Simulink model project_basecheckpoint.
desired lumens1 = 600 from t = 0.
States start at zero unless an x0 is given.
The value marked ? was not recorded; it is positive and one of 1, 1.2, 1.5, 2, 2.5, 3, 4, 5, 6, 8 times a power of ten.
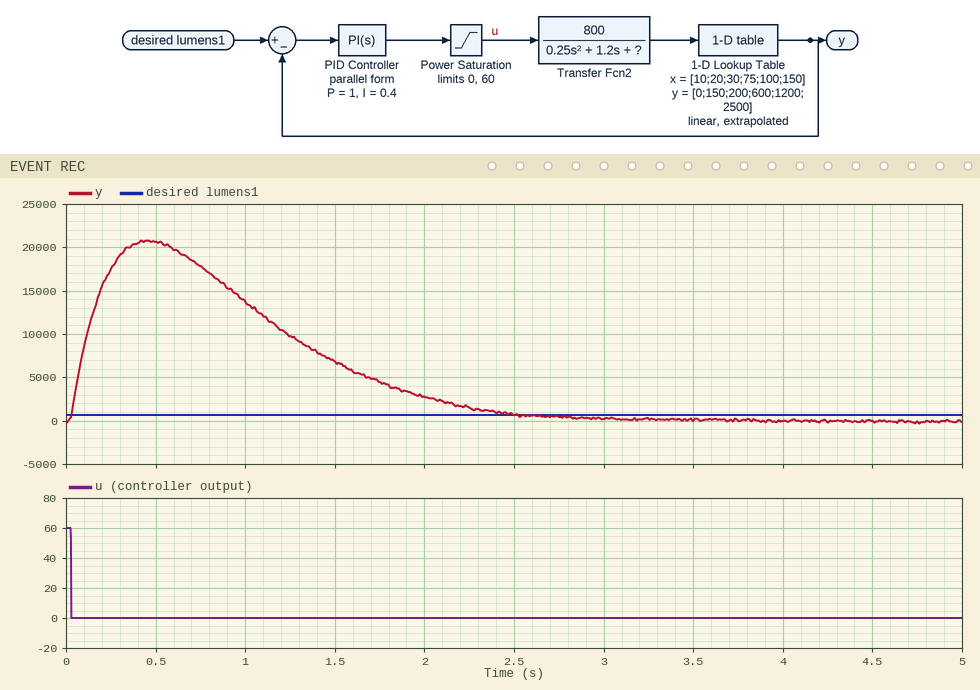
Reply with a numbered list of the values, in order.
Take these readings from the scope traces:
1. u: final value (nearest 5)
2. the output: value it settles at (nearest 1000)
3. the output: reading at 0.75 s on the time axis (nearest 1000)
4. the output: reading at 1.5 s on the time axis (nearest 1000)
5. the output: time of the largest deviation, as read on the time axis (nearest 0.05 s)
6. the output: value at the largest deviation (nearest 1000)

1. 0
2. 0
3. 18000
4. 7000
5. 0.45 s
6. 21000
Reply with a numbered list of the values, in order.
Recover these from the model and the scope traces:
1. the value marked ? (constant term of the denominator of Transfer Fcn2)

1. 1.2
